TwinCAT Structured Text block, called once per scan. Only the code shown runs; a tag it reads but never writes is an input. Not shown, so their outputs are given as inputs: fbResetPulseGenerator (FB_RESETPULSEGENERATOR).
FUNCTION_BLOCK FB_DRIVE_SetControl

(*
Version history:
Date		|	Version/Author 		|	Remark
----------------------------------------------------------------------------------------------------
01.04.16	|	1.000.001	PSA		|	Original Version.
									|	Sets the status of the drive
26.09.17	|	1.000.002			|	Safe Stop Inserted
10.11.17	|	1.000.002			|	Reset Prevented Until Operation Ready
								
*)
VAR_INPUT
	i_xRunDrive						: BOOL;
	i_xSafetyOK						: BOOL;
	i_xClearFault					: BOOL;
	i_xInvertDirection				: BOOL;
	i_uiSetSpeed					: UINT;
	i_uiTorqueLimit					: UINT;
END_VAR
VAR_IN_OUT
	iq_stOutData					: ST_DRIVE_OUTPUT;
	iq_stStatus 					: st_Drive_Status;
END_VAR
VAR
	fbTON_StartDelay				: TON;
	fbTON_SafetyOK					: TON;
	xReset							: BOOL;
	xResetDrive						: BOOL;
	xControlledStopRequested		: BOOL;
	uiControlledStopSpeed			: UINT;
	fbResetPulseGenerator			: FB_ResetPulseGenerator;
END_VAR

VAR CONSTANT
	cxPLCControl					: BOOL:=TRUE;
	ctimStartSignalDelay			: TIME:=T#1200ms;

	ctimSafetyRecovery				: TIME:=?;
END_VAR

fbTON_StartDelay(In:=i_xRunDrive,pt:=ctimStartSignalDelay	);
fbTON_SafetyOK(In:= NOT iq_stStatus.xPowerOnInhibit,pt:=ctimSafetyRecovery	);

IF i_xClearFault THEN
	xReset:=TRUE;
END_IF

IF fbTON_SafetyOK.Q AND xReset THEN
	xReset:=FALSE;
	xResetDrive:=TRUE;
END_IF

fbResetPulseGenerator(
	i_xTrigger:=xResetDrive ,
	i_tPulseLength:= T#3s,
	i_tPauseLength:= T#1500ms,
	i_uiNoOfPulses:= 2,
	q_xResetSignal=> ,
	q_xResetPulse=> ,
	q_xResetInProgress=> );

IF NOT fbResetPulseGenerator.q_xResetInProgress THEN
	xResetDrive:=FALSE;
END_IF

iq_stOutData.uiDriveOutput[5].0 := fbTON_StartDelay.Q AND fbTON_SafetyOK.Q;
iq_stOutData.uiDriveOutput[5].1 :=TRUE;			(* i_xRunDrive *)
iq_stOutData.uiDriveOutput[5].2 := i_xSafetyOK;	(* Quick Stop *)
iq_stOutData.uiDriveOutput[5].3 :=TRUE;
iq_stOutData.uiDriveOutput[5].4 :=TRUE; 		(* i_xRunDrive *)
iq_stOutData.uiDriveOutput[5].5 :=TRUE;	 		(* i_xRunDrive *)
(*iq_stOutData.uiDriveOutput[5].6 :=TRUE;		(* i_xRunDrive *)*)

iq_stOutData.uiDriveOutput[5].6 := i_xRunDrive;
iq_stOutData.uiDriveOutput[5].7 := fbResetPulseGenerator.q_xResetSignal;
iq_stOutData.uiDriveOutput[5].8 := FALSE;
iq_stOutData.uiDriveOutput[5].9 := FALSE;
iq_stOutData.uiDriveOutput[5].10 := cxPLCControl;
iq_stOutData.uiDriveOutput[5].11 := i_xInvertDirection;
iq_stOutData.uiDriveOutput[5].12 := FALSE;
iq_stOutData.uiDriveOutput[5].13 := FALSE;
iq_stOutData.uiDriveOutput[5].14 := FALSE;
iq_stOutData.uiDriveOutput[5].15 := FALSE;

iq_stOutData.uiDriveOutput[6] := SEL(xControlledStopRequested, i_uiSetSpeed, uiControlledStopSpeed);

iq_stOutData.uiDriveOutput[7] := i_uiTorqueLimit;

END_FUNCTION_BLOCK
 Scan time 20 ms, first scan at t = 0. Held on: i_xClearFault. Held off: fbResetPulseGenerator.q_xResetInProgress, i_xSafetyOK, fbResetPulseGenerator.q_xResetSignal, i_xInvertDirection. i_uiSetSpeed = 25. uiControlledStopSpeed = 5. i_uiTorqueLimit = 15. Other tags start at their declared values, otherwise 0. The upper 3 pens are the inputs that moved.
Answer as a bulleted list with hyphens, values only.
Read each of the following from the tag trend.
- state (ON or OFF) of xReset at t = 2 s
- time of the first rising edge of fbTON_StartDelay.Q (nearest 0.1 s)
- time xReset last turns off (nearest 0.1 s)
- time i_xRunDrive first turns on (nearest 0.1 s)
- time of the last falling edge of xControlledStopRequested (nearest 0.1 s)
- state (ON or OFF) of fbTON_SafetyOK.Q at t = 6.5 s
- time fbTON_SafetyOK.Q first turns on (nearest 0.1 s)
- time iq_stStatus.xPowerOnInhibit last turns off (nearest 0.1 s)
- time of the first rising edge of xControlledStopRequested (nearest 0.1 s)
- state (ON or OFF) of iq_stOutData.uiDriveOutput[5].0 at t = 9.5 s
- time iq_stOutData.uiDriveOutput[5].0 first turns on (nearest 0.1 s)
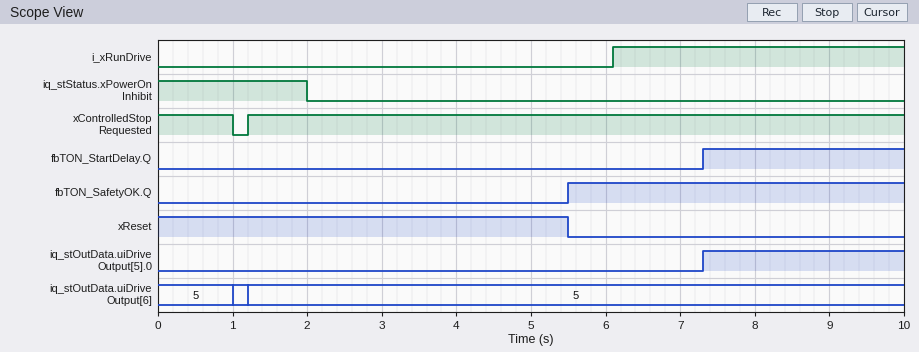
- ON
- 7.3 s
- 5.5 s
- 6.1 s
- 1.0 s
- ON
- 5.5 s
- 2.0 s
- 1.2 s
- ON
- 7.3 s
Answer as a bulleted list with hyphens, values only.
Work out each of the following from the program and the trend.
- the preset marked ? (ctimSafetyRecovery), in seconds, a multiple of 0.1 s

- 3.5 s
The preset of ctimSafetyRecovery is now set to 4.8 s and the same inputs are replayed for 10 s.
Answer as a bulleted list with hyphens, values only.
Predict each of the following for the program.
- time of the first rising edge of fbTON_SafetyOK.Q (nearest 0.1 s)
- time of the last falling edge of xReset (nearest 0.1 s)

- 6.8 s
- 6.8 s
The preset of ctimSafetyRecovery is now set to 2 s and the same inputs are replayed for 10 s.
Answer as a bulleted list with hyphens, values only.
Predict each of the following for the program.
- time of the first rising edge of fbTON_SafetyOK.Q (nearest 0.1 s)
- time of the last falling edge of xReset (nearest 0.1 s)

- 4.0 s
- 4.0 s
